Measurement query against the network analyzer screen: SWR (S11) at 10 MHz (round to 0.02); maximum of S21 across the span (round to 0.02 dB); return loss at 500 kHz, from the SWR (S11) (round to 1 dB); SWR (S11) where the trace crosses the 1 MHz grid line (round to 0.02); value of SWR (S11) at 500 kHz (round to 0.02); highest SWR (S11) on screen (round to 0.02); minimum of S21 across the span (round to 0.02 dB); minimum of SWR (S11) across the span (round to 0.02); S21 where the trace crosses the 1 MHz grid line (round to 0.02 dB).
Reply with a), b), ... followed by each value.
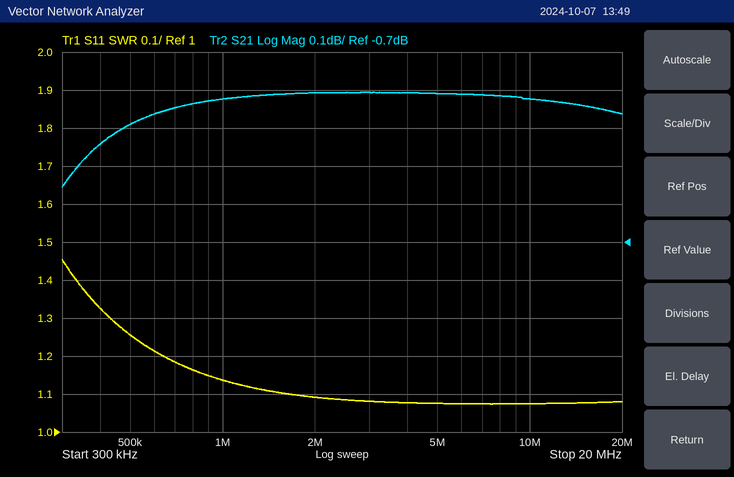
a) 1.08
b) -0.30 dB
c) 19 dB
d) 1.14
e) 1.26
f) 1.46
g) -0.56 dB
h) 1.08
i) -0.32 dB
